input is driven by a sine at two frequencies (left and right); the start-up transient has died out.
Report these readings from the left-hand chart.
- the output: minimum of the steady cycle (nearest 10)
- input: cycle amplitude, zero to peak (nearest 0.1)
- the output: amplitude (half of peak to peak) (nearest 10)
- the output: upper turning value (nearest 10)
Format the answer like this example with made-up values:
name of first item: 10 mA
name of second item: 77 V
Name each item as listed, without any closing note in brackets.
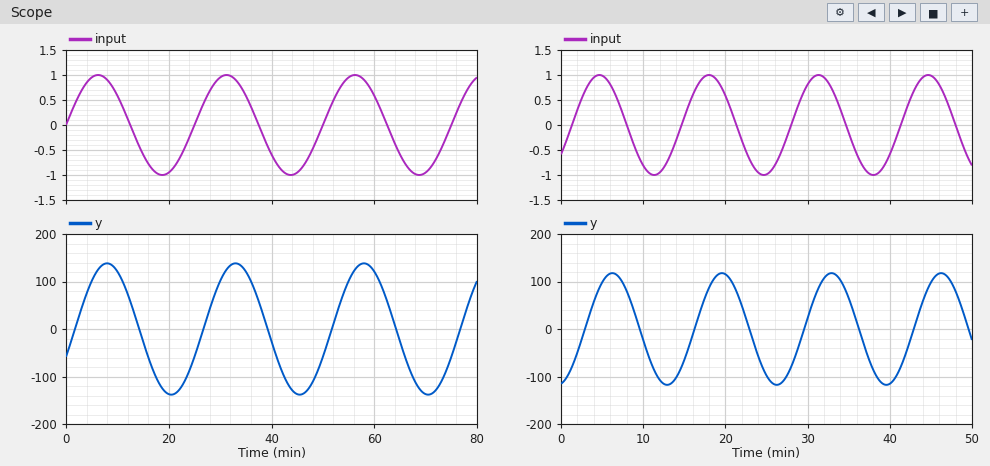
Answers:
the output: minimum of the steady cycle: -140
input: cycle amplitude, zero to peak: 1.0
the output: amplitude (half of peak to peak): 140
the output: upper turning value: 140
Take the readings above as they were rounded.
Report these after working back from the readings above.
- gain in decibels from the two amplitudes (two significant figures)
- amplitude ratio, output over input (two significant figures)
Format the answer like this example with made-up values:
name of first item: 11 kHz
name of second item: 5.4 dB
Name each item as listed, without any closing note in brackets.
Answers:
gain in decibels from the two amplitudes: 43 dB
amplitude ratio, output over input: 140
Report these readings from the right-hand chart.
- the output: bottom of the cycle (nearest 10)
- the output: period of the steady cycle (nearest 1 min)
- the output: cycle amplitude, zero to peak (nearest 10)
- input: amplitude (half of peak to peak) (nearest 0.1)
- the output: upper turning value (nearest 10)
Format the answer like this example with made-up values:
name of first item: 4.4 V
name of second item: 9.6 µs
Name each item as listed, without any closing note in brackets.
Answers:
the output: bottom of the cycle: -120
the output: period of the steady cycle: 13 min
the output: cycle amplitude, zero to peak: 120
input: amplitude (half of peak to peak): 1.0
the output: upper turning value: 120
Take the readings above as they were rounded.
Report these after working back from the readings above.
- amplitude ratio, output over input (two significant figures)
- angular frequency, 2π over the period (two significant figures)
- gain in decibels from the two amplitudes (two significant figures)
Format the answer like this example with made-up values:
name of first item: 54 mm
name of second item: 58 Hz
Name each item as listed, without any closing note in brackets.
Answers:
amplitude ratio, output over input: 120
angular frequency, 2π over the period: 0.48 rad/min
gain in decibels from the two amplitudes: 42 dB
